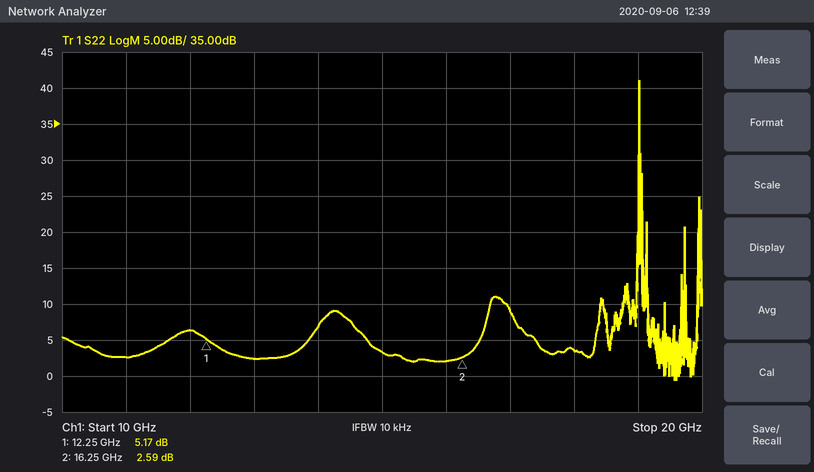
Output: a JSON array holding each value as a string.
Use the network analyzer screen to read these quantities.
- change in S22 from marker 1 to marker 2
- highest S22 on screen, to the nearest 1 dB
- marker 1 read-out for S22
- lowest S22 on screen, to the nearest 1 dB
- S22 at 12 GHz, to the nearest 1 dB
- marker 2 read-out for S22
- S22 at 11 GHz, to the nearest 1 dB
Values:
["-2.58 dB", "41 dB", "5.17 dB", "-1 dB", "6 dB", "2.59 dB", "3 dB"]
